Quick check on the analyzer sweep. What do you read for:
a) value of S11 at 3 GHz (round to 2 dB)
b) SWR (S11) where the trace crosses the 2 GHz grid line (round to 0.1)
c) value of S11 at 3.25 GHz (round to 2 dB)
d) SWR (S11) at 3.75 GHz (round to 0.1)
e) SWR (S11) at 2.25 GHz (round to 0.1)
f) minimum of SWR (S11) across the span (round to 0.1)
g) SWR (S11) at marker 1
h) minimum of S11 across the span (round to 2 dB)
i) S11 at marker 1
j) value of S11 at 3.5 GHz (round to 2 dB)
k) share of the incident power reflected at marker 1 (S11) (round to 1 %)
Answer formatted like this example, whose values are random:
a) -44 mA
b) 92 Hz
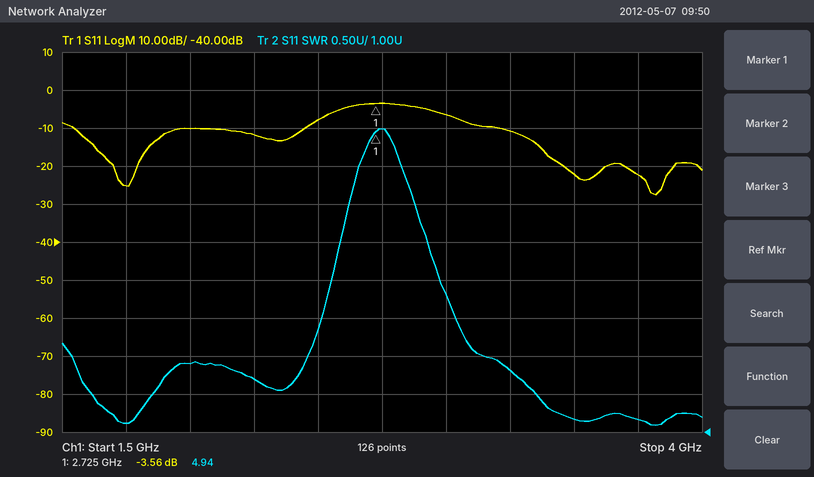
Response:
a) -6 dB
b) 1.9
c) -10 dB
d) 1.2
e) 1.7
f) 1.1
g) 4.94
h) -28 dB
i) -3.56 dB
j) -22 dB
k) 44 %
